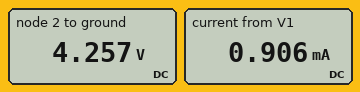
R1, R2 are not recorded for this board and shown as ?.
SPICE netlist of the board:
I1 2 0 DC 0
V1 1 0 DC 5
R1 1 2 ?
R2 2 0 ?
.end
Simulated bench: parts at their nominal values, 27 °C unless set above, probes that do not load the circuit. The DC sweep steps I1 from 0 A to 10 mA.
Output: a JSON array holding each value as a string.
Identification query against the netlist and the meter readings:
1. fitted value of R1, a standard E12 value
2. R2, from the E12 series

["820 Ω", "4.7 kΩ"]
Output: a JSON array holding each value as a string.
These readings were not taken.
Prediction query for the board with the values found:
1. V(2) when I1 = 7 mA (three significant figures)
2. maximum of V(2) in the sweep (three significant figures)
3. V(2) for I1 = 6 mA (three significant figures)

["-630 mV", "4.26 V", "68.1 mV"]
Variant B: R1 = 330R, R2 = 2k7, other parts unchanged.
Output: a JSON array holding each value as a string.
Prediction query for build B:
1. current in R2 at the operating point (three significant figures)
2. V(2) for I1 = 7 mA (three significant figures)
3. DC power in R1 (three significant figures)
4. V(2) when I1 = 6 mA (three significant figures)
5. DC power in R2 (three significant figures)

["1.65 mA", "2.40 V", "899 µW", "2.69 V", "7.35 mW"]
